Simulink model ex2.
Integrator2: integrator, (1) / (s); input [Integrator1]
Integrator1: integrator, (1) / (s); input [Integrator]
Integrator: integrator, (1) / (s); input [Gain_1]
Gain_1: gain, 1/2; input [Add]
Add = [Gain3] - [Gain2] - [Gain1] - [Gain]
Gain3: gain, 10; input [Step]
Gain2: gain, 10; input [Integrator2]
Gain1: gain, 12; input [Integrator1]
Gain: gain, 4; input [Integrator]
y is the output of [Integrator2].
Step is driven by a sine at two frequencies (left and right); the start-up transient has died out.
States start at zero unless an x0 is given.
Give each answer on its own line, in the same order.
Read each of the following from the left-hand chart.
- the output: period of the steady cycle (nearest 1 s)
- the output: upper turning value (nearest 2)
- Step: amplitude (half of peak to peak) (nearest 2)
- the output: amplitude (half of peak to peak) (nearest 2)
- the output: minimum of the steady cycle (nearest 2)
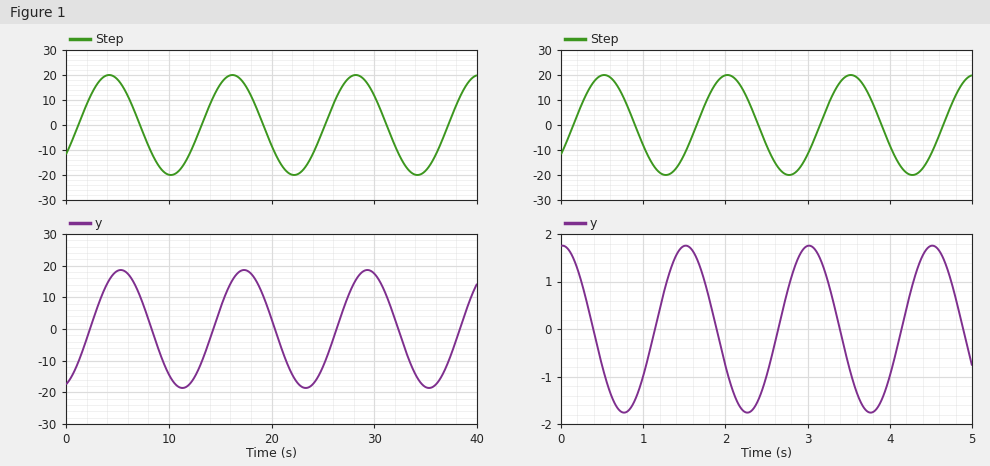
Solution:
12 s
18
20
18
-18
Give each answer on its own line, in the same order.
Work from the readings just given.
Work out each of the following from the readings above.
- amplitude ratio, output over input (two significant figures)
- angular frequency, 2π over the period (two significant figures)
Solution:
0.90
0.52 rad/s
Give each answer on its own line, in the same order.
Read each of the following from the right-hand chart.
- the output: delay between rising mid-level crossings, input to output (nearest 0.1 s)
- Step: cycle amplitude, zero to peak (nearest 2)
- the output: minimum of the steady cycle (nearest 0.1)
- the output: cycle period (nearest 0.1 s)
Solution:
1.0 s
20
-1.8
1.5 s
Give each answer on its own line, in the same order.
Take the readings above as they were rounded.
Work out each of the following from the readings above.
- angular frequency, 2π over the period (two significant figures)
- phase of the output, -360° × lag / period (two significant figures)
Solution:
4.2 rad/s
-240°
